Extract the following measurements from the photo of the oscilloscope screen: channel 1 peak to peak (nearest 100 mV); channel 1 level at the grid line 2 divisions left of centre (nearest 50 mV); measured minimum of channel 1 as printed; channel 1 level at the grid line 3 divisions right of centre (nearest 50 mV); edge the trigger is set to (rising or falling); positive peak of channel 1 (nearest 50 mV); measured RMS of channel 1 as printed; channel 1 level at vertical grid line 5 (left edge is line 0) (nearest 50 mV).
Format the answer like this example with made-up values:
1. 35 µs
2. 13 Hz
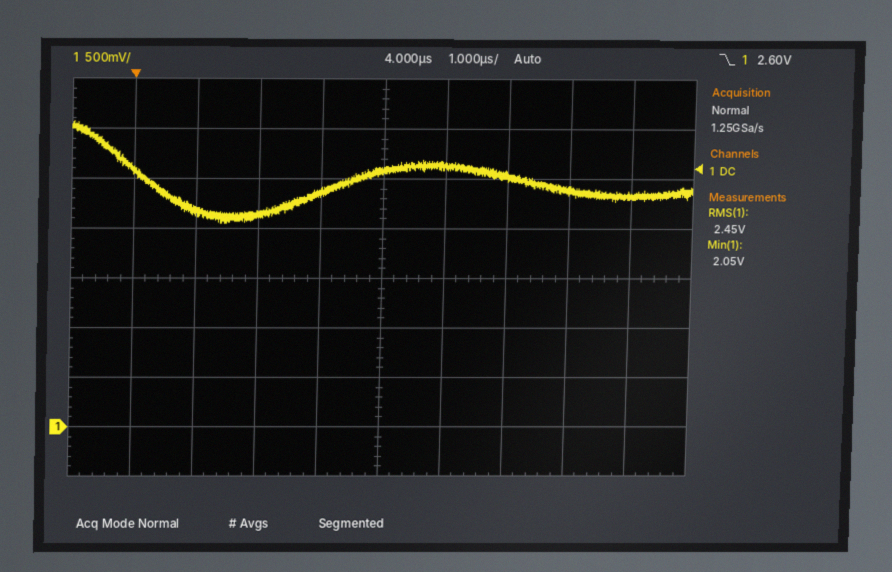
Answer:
1. 1.00 V
2. 2.15 V
3. 2.05 V
4. 2.40 V
5. falling
6. 3.05 V
7. 2.45 V
8. 2.60 V
